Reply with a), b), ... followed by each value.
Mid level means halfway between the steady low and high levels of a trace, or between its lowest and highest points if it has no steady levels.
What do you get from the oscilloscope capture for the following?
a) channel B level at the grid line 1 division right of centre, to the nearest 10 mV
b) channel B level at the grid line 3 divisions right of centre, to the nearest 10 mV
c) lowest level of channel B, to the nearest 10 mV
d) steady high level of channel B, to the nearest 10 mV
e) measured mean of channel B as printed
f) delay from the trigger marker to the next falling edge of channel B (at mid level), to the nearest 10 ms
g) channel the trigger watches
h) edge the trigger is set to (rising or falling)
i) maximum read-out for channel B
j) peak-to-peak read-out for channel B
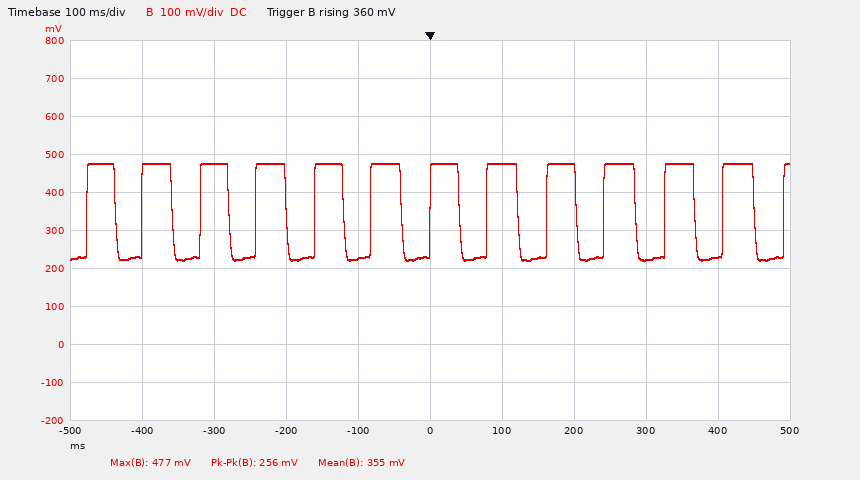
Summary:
a) 480 mV
b) 220 mV
c) 220 mV
d) 480 mV
e) 355 mV
f) 40 ms
g) channel B
h) rising
i) 477 mV
j) 256 mV
